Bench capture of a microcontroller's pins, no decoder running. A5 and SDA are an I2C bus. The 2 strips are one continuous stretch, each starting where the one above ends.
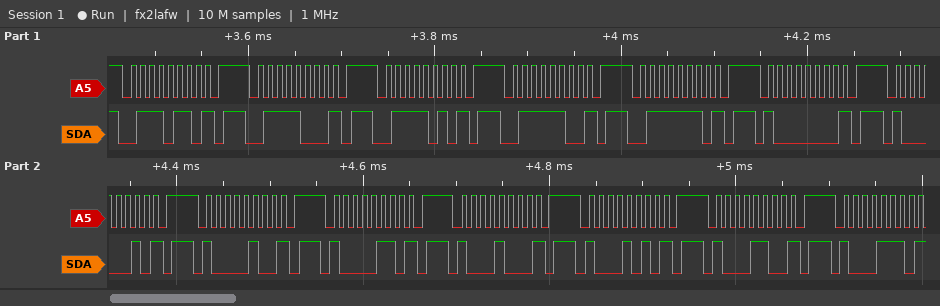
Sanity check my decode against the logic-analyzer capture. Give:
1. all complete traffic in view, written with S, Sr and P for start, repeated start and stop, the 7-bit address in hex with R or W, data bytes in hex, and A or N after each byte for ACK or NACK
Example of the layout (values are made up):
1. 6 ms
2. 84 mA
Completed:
1. S 3BW N P S 3CW N P S 3DW N P S 3EW N P S 3FW N P S 40W N P S 41W N P S 42W N P S 43W N P S 44W N P S 45W N P S 46W N P S 47W N
